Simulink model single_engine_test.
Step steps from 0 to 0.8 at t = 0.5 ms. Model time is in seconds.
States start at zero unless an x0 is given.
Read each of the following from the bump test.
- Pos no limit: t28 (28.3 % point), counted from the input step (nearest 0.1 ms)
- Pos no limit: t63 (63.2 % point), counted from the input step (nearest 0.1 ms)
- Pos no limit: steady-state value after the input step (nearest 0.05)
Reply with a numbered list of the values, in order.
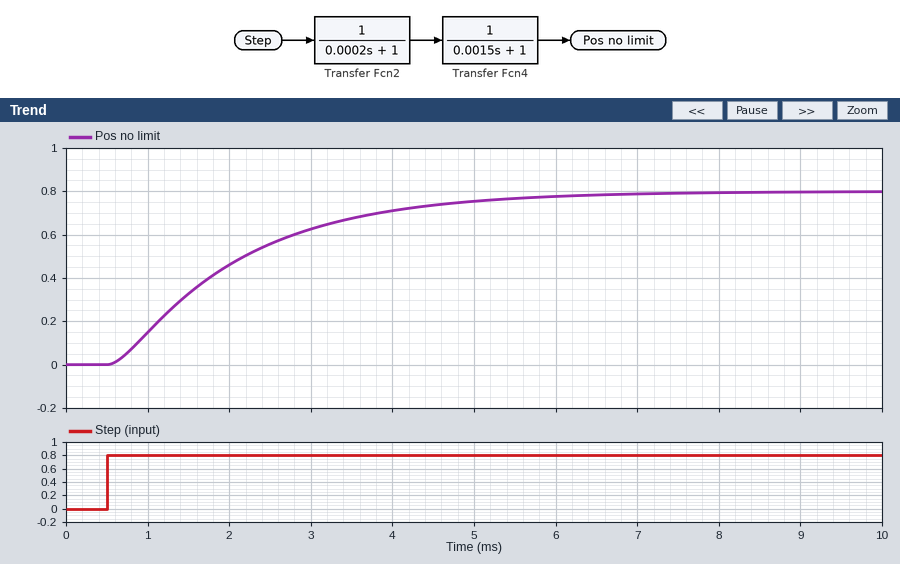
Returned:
1. 0.7 ms
2. 1.7 ms
3. 0.80
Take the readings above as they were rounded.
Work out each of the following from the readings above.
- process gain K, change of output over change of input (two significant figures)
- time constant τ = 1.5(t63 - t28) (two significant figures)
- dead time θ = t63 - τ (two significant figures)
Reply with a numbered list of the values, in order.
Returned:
1. 1.0
2. 1.5 ms
3. 0.20 ms
